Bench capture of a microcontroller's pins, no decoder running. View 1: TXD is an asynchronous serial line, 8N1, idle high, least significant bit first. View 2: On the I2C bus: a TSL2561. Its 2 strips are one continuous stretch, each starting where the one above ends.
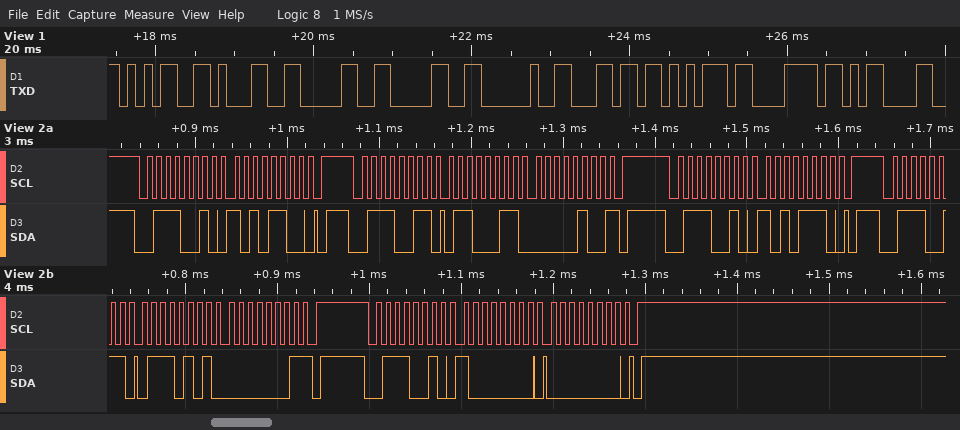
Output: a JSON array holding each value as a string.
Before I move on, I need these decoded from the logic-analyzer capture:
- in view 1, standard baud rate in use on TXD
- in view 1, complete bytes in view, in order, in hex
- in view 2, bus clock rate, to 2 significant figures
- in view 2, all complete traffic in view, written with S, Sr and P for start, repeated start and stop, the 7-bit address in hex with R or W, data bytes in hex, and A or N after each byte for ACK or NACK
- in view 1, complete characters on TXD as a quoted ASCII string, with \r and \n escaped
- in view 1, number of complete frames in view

["9600 baud", "0x35 0x31 0x30 0x30 0x20 0x6C 0x75 0x78 0x0D", "100 kHz", "S 39W A AC A P S 39R A 63 A 04 N P S 39W A AE A P S 39R A 75 A 01 N P S 39W A 80 A 00 A P", "\"5100 lux\\r\"", "9"]
